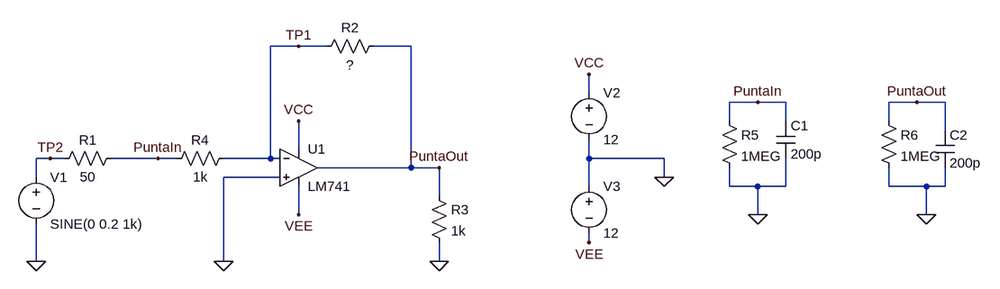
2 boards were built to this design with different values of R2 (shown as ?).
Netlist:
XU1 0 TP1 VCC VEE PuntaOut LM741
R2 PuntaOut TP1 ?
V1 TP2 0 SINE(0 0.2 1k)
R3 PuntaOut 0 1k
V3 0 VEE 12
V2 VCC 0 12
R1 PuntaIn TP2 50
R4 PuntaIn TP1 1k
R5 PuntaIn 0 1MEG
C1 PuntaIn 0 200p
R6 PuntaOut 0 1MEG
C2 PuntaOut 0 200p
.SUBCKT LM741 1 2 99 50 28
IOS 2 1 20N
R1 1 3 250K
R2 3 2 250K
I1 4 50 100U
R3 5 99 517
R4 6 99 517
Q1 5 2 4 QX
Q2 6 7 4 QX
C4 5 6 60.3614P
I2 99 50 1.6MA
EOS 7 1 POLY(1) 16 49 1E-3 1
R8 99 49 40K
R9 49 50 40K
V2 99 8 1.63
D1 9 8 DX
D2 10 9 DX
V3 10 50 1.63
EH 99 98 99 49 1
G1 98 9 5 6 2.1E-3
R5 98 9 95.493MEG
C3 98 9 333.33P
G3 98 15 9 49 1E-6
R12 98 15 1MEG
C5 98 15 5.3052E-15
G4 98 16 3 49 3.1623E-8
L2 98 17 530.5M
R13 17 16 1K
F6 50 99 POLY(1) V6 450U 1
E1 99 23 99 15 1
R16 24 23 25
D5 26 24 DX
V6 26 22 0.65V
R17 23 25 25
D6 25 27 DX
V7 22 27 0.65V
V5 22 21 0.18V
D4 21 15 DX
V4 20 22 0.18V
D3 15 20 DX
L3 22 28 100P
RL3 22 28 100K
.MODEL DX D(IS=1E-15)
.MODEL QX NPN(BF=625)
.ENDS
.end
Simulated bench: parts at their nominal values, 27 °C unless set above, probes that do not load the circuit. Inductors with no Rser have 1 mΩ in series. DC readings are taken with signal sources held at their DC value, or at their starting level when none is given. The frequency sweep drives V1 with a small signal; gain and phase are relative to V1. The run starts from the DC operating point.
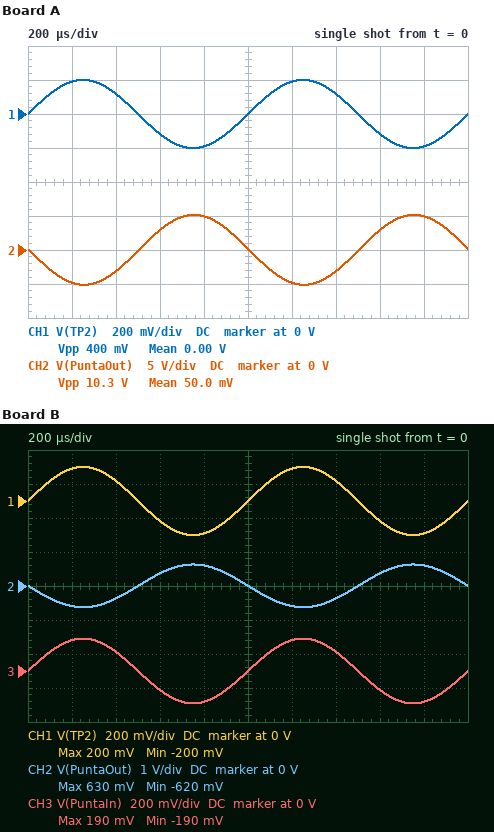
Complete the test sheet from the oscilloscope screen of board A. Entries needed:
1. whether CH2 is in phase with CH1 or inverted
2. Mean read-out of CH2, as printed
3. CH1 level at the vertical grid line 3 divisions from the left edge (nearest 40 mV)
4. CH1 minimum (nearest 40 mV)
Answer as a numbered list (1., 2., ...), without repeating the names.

1. inverted
2. 50.0 mV
3. -120 mV
4. -200 mV
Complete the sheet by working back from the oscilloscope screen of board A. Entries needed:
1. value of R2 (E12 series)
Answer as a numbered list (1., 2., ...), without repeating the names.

1. 27 kΩ
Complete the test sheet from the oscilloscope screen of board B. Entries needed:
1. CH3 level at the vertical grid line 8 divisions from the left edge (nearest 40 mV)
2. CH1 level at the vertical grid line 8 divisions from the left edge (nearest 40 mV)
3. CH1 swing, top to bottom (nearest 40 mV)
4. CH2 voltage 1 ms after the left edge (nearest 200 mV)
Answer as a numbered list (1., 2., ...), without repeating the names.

1. -120 mV
2. -120 mV
3. 400 mV
4. 0 V
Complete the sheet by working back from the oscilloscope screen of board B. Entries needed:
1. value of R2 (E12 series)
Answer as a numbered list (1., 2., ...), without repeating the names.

1. 3.3 kΩ
